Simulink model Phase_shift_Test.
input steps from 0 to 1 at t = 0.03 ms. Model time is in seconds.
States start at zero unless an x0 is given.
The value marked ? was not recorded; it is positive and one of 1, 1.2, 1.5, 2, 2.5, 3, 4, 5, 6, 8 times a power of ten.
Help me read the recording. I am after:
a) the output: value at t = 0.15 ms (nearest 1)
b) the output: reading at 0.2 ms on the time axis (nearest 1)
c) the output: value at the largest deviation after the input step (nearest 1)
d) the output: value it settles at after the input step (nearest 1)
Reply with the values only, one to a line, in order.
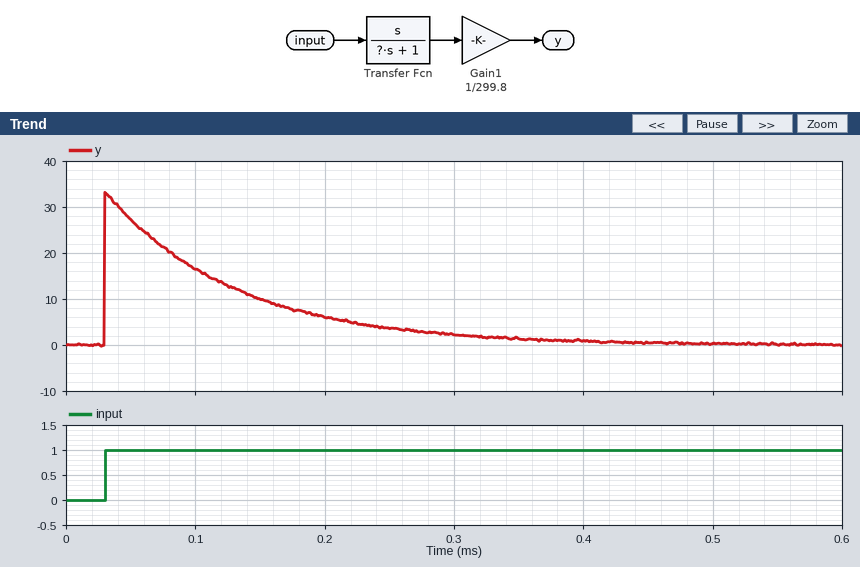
10
6
33
0
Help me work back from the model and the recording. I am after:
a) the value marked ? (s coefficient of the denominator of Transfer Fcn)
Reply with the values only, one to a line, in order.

0.0001
